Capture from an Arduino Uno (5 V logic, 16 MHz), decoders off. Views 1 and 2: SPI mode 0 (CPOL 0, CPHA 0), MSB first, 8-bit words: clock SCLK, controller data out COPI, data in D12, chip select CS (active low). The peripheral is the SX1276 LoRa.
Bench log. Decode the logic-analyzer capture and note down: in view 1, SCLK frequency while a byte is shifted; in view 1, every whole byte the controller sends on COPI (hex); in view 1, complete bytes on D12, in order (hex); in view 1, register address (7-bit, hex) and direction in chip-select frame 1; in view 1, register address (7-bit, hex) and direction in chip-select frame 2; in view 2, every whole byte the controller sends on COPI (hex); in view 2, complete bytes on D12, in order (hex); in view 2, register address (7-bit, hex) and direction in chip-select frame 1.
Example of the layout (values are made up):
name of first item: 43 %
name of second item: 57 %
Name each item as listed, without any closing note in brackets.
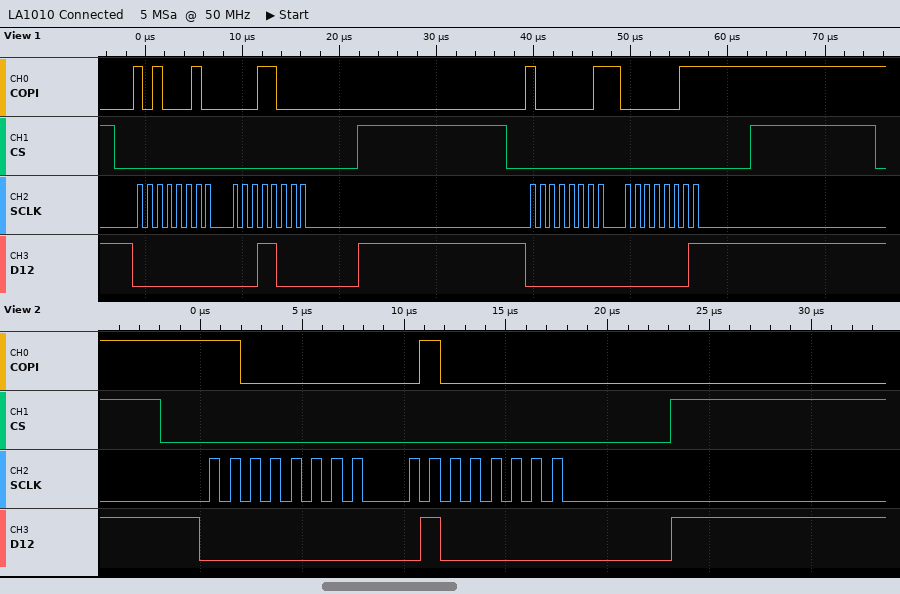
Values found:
in view 1, SCLK frequency while a byte is shifted: 1 MHz
in view 1, every whole byte the controller sends on COPI: A2 18 81 03
in view 1, complete bytes on D12, in order: 00 18 00 01
in view 1, register address (7-bit, hex) and direction in chip-select frame 1: 0x22 write
in view 1, register address (7-bit, hex) and direction in chip-select frame 2: 0x01 write
in view 2, every whole byte the controller sends on COPI: 0xC0 0x40
in view 2, complete bytes on D12, in order: 0x00 0x40
in view 2, register address (7-bit, hex) and direction in chip-select frame 1: 0x40 write
